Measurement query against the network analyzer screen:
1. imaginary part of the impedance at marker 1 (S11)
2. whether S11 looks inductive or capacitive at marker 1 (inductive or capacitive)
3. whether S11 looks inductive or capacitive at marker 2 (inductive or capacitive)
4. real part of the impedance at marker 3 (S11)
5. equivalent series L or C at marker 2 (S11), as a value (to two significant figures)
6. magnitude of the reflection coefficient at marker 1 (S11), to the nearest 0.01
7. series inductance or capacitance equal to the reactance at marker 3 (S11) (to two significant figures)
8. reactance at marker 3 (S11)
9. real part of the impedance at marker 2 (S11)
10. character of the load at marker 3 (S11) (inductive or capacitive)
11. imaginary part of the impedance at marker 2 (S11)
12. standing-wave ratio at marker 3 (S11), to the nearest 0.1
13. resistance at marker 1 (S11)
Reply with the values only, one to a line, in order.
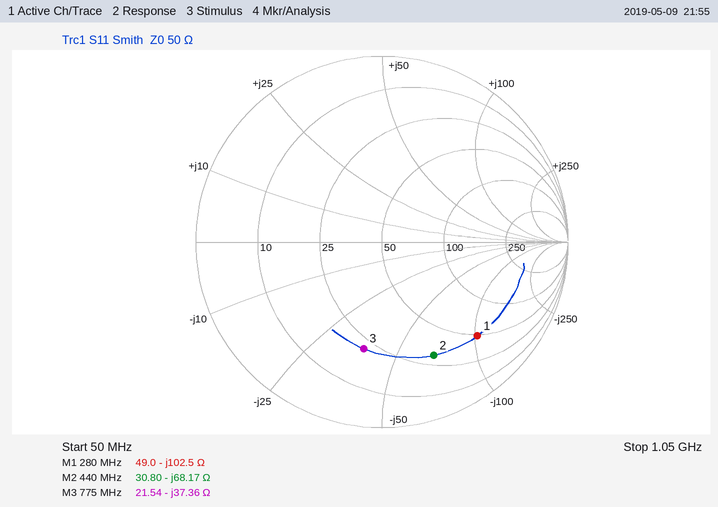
-102.5 Ω
capacitive
capacitive
21.54 Ω
5.3 pF
0.72
5.5 pF
-37.36 Ω
30.80 Ω
capacitive
-68.17 Ω
3.8
49.0 Ω
